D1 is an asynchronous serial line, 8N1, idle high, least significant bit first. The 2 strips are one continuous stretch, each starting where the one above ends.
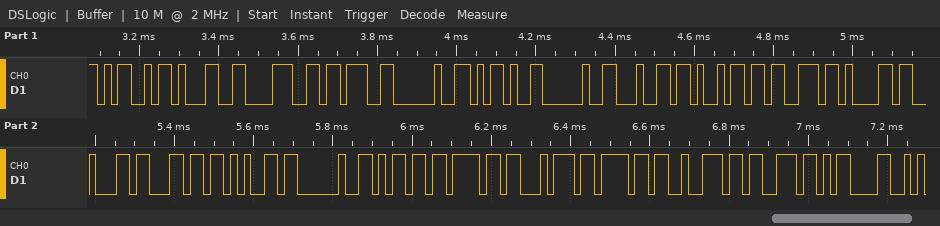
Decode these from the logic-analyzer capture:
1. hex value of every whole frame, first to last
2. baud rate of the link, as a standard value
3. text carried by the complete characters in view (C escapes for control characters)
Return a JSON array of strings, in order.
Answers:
["4D 31 38 3B 20 2D 20 64 69 73 61 62 6C 65 20 6D 6F 74 6F 72 73 0D", "57600 baud", "\"M18; - disable motors\\r\""]
